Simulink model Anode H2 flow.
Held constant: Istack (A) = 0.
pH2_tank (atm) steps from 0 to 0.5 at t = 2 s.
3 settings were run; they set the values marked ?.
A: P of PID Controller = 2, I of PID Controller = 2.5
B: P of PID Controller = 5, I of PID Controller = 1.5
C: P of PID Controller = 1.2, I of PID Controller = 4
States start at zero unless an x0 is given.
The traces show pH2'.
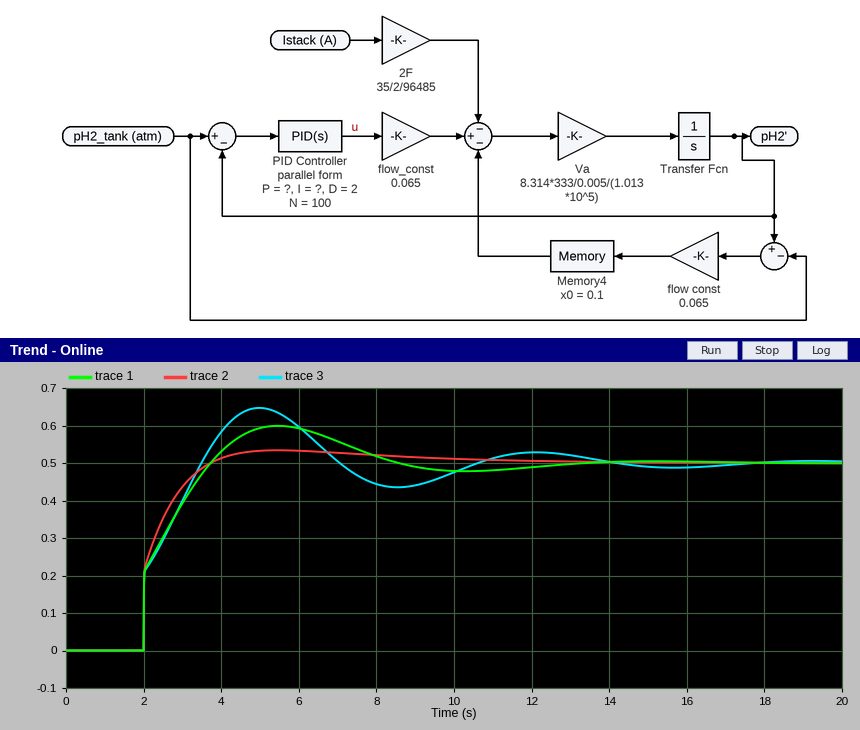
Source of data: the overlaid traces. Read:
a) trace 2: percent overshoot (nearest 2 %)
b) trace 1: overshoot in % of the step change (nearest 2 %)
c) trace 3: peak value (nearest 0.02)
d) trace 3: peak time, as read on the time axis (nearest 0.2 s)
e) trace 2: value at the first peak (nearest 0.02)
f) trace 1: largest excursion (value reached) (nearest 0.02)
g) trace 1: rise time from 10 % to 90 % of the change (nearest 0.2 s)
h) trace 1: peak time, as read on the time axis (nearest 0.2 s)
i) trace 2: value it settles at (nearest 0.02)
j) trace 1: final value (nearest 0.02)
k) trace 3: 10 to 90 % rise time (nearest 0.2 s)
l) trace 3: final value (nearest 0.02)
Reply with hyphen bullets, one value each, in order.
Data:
- 6 %
- 20 %
- 0.64
- 5.0 s
- 0.54
- 0.60
- 1.4 s
- 5.4 s
- 0.50
- 0.50
- 1.2 s
- 0.50
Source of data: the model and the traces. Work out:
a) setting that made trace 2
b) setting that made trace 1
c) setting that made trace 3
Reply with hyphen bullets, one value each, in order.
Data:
- B
- A
- C
